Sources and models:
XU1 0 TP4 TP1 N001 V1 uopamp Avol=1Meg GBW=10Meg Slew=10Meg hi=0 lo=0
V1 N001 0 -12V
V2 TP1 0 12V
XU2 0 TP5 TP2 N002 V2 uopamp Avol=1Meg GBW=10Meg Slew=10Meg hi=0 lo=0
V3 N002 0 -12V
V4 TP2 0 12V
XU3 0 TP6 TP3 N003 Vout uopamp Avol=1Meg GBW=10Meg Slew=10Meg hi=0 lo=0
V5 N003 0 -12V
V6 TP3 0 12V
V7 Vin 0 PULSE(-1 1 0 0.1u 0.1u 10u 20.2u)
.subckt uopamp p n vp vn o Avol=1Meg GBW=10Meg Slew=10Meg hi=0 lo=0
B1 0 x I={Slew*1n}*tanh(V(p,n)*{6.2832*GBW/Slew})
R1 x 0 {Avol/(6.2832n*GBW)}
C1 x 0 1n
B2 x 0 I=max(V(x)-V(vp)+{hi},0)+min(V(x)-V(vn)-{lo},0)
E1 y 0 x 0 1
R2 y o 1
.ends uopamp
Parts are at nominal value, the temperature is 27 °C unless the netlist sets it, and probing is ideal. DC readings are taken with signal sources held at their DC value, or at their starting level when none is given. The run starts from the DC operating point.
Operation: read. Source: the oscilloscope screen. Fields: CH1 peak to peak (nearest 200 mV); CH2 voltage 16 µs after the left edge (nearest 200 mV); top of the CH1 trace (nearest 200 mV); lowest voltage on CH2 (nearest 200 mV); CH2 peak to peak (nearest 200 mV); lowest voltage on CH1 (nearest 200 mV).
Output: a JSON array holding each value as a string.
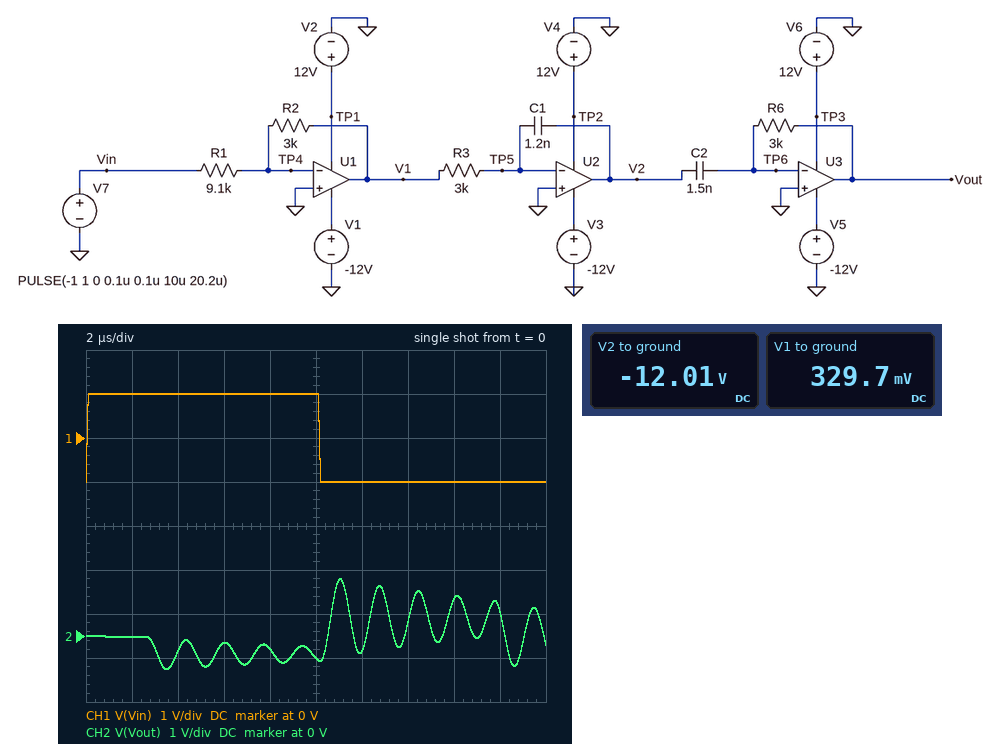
["2.0 V", "800 mV", "1.0 V", "-800 mV", "2.0 V", "-1.0 V"]
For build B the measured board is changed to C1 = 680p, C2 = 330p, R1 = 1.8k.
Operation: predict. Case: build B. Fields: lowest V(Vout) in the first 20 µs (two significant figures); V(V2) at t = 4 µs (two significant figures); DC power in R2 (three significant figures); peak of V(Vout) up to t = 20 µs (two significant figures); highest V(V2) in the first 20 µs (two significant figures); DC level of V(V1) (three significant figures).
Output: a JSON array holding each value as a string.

["-1.4 V", "-10 V", "926 µW", "1.7 V", "-5.0 V", "1.67 V"]
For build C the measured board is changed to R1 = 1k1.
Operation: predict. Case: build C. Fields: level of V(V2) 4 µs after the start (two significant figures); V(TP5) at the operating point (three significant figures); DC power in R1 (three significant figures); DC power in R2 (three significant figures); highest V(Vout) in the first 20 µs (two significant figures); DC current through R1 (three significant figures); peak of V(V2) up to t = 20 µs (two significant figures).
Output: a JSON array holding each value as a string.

["-11 V", "2.73 V", "909 µW", "2.48 mW", "7.6 V", "909 µA", "-6.4 V"]
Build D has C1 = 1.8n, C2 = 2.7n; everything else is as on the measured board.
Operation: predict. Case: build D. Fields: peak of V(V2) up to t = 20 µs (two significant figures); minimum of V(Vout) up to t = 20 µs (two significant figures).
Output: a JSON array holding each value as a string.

["-12 V", "-920 mV"]
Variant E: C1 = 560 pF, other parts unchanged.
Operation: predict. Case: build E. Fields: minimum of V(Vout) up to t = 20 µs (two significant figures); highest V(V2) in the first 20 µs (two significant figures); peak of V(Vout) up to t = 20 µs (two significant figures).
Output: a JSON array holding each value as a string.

["-1.6 V", "-10 V", "2.5 V"]
